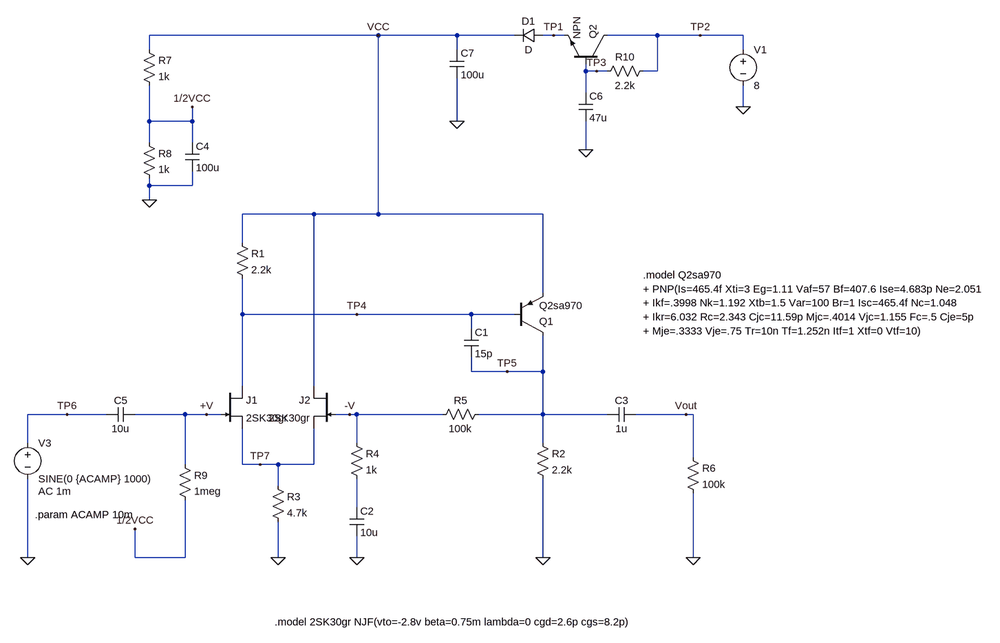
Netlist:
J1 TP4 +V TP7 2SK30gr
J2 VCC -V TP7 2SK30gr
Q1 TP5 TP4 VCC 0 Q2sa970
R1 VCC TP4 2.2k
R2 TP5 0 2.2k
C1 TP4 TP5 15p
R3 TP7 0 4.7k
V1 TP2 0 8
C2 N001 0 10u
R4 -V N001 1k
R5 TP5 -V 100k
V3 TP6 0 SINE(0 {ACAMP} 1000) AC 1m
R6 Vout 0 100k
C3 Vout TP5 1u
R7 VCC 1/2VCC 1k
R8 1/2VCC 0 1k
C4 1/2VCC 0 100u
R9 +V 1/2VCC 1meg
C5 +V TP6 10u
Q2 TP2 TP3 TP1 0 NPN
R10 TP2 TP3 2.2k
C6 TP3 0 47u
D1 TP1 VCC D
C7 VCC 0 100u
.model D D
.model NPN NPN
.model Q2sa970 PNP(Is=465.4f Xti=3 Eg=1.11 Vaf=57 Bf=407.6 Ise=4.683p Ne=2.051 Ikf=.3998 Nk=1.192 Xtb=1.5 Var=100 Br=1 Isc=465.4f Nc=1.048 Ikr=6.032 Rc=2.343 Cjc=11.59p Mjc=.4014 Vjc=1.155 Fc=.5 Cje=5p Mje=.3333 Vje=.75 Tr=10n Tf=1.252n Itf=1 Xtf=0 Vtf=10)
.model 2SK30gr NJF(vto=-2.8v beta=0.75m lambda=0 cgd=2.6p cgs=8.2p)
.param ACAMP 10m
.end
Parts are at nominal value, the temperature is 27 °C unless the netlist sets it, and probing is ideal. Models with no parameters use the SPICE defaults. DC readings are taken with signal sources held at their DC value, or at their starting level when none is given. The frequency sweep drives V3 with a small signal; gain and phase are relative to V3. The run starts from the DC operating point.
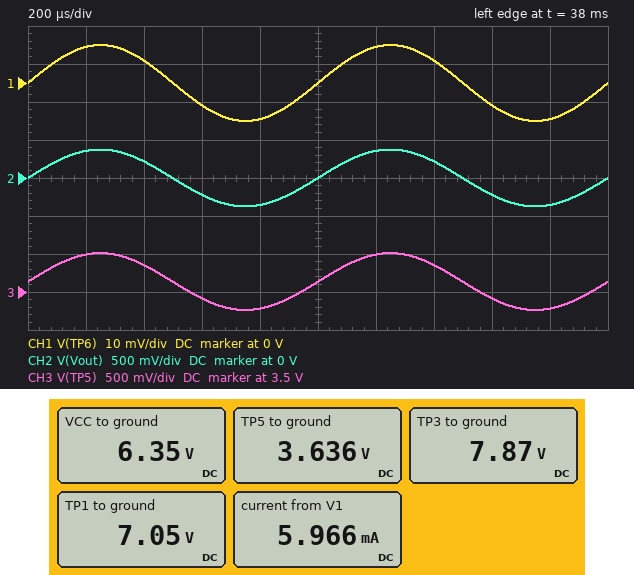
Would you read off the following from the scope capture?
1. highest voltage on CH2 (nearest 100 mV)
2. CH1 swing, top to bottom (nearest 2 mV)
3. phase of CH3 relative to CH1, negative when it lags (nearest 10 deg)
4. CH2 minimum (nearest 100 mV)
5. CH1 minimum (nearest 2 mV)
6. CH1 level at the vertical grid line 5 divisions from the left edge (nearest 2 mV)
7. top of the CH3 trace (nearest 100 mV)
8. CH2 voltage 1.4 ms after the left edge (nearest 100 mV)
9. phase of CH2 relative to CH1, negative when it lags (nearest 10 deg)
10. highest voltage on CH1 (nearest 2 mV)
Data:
400 mV
20 mV
0 deg
-400 mV
-10 mV
0 V
4.0 V
200 mV
0 deg
10 mV
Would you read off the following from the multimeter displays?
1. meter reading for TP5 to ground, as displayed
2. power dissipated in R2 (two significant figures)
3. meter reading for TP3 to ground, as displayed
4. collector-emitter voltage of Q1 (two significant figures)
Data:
3.636 V
6.0 mW
7.87 V
-2.7 V
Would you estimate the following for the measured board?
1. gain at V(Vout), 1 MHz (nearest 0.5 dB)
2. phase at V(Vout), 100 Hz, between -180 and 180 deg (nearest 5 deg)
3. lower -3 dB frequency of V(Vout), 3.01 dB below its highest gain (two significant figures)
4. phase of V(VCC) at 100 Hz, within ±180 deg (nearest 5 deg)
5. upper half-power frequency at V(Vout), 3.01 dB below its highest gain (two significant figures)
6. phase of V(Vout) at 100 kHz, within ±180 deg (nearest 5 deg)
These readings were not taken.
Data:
9.0 dB
5 deg
8.1 Hz
155 deg
76 kHz
-55 deg
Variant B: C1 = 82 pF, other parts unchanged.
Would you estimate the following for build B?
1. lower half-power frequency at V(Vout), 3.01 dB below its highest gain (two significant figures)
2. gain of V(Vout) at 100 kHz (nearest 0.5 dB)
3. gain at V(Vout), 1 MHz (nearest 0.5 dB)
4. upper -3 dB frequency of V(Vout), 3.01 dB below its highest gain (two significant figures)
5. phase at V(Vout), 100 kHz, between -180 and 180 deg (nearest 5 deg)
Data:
8.0 Hz
17.0 dB
-2.5 dB
20 kHz
-80 deg
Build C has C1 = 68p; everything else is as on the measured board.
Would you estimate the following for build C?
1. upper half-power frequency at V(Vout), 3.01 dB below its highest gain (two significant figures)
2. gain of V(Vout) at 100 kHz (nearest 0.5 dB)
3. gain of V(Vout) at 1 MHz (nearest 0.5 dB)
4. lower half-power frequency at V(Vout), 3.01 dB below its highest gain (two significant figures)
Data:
23 kHz
18.5 dB
-1.0 dB
8.0 Hz
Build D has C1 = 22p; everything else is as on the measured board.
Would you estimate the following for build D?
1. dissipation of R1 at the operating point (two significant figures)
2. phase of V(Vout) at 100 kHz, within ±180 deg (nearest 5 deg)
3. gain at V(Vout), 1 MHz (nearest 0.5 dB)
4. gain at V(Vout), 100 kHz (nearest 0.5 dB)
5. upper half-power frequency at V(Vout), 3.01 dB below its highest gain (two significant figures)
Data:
150 µW
-60 deg
7.0 dB
25.5 dB
59 kHz
